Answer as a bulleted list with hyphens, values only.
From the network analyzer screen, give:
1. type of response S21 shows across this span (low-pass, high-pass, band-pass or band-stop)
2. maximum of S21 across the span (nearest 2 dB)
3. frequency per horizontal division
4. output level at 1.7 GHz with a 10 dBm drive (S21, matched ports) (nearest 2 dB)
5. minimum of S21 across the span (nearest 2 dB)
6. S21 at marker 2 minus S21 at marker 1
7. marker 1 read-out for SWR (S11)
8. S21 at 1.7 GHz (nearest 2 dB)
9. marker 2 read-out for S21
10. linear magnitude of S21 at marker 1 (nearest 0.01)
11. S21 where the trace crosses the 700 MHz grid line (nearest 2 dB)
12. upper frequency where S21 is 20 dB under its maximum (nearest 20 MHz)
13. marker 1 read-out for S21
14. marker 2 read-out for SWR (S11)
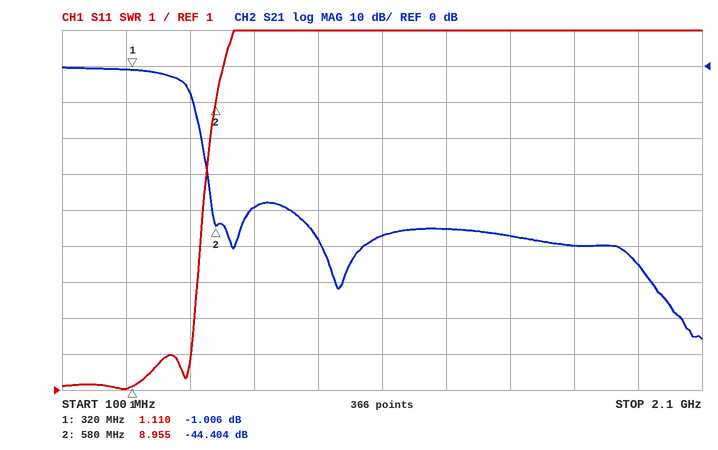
- low-pass
- 0 dB
- 200 MHz
- -40 dBm
- -76 dB
- -43.398 dB
- 1.110
- -50 dB
- -44.404 dB
- 0.89
- -40 dB
- 540 MHz
- -1.006 dB
- 8.955
